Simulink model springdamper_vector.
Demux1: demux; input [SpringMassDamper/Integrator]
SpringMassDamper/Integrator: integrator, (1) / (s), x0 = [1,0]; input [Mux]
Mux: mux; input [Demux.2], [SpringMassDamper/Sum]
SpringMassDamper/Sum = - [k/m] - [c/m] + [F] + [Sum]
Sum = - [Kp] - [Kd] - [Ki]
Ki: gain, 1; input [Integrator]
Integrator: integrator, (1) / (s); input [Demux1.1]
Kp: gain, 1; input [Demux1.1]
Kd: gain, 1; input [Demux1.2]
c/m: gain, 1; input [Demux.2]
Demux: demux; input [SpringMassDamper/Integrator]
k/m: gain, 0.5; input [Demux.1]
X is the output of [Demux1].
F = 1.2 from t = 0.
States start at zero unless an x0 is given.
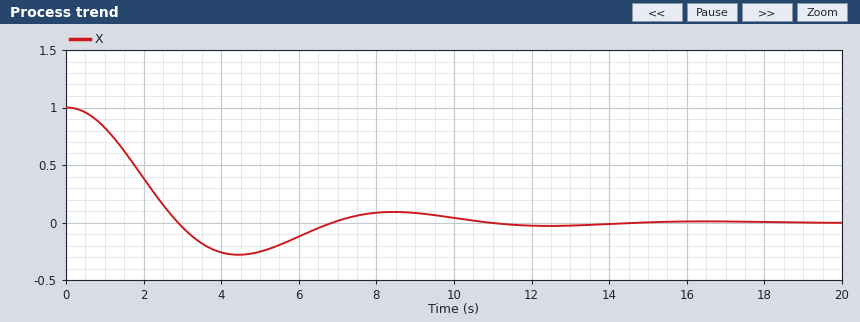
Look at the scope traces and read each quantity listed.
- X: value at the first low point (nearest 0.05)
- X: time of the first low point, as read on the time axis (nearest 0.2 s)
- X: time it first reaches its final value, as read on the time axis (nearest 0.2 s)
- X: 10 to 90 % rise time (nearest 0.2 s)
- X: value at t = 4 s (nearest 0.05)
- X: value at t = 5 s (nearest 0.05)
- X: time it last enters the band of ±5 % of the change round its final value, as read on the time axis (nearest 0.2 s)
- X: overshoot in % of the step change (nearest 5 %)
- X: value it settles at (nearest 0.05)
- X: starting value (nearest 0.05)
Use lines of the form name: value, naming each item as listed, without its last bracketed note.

X: value at the first low point: -0.30
X: time of the first low point, as read on the time axis: 4.4 s
X: time it first reaches its final value, as read on the time axis: 2.8 s
X: 10 to 90 % rise time: 1.8 s
X: value at t = 4 s: -0.25
X: value at t = 5 s: -0.25
X: time it last enters the band of ±5 % of the change round its final value, as read on the time axis: 9.8 s
X: overshoot in % of the step change: 30 %
X: value it settles at: 0.00
X: starting value: 1.00
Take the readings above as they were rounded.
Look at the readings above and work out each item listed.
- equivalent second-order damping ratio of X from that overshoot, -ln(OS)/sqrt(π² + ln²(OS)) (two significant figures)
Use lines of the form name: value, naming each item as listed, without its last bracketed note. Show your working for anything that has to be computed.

equivalent second-order damping ratio of X from that overshoot, -ln(OS)/sqrt(π² + ln²(OS)): ln(0.3) = -1.204; 1.204 / sqrt(9.870 + 1.450) = 0.36
